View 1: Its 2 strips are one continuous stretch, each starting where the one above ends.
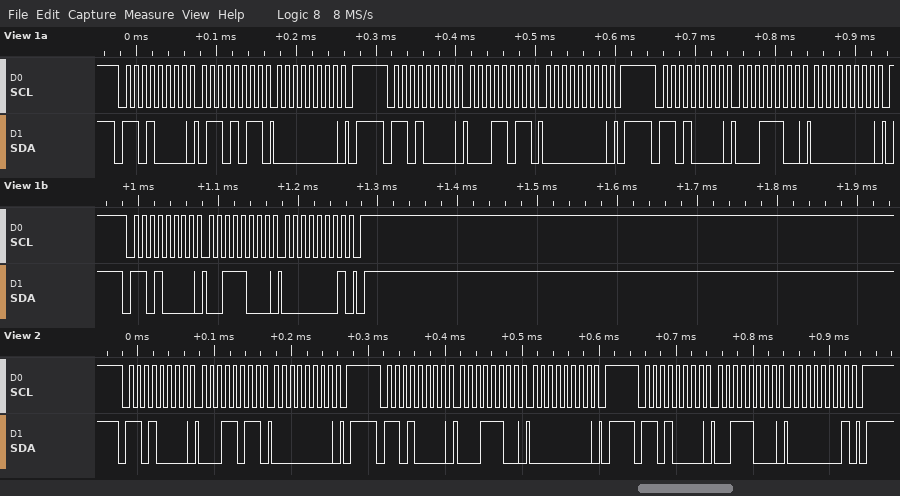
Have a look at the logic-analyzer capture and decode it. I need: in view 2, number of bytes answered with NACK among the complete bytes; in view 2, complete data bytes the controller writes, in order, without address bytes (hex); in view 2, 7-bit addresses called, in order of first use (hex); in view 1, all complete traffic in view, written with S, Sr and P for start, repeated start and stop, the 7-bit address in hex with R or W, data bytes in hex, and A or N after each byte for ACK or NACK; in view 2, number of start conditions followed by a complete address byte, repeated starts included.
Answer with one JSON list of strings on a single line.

["0", "1B 00 1C 00 38 01", "0x68", "S 68W A 6B A 00 A P S 68W A 1B A 00 A P S 68W A 1C A 00 A P S 68W A 38 A 01 A P", "3"]
